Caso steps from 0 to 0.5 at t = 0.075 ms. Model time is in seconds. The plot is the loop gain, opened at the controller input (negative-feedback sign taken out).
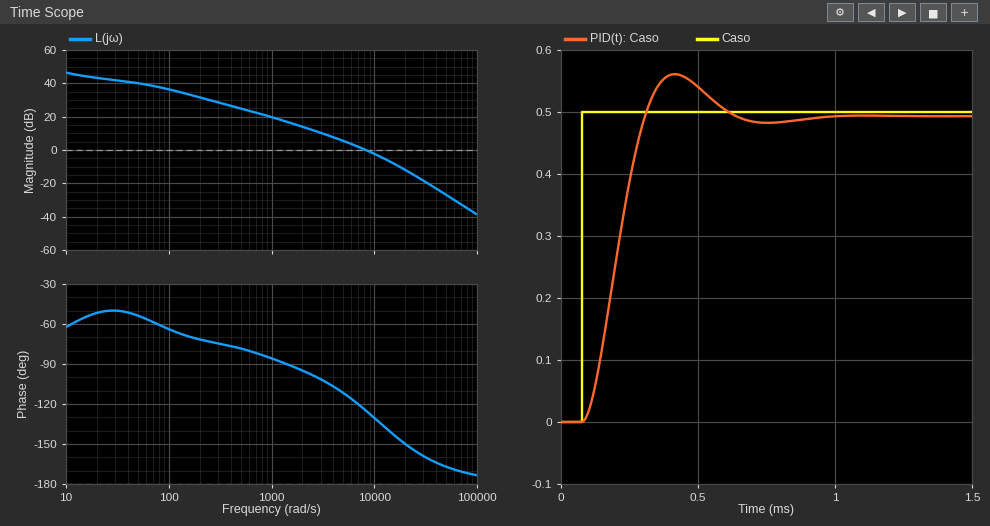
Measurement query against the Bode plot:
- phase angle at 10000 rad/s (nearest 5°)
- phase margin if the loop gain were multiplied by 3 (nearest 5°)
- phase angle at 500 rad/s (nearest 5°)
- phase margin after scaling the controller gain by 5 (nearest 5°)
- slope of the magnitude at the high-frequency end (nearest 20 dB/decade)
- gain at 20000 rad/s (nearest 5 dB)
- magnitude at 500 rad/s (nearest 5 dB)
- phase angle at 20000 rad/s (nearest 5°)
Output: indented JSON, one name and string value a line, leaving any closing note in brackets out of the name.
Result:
{
  "phase angle at 10000 rad/s": "-130°",
  "phase margin if the loop gain were multiplied by 3": "35°",
  "phase angle at 500 rad/s": "-80°",
  "phase margin after scaling the controller gain by 5": "25°",
  "slope of the magnitude at the high-frequency end": "-40 dB/decade",
  "gain at 20000 rad/s": "-10 dB",
  "magnitude at 500 rad/s": "25 dB",
  "phase angle at 20000 rad/s": "-150°"
}
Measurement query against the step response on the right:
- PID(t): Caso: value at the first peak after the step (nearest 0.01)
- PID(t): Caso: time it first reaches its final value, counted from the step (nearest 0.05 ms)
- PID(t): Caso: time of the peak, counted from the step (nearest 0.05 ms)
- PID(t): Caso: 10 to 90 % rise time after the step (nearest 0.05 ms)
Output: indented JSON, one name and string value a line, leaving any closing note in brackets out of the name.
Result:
{
  "PID(t): Caso: value at the first peak after the step": "0.56",
  "PID(t): Caso: time it first reaches its final value, counted from the step": "0.25 ms",
  "PID(t): Caso: time of the peak, counted from the step": "0.35 ms",
  "PID(t): Caso: 10 to 90 % rise time after the step": "0.15 ms"
}
